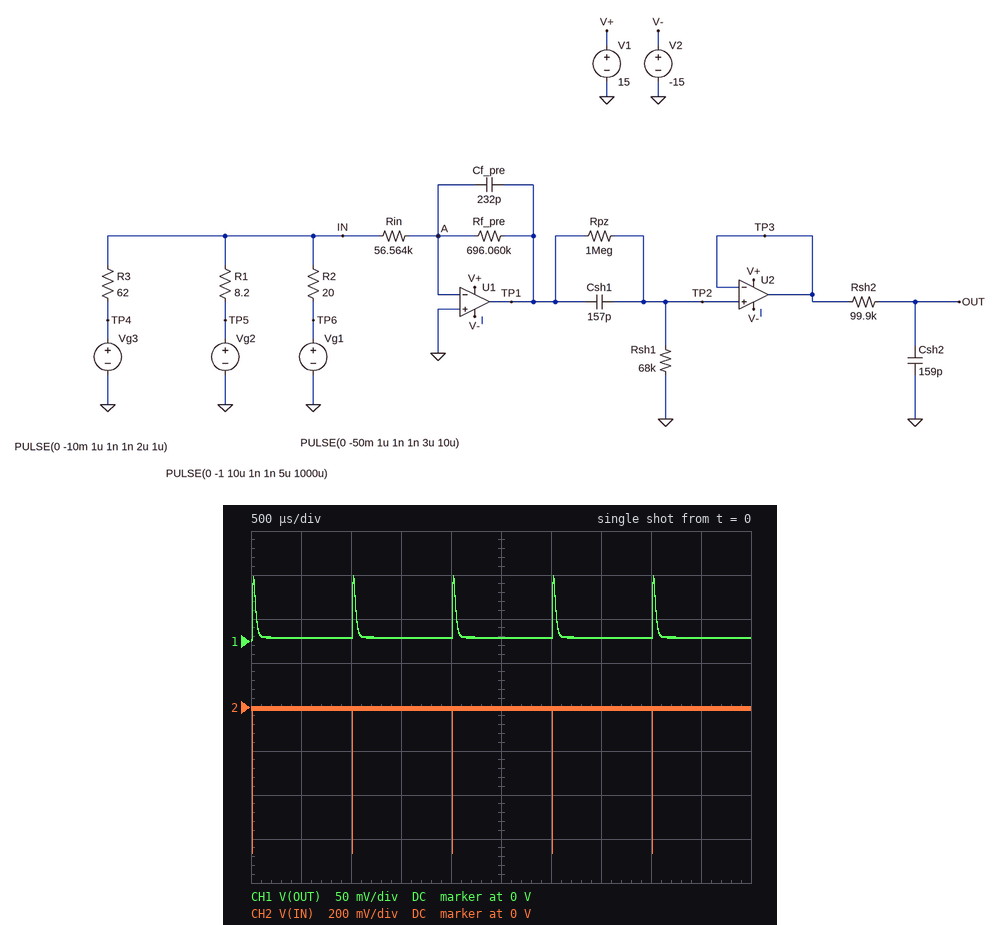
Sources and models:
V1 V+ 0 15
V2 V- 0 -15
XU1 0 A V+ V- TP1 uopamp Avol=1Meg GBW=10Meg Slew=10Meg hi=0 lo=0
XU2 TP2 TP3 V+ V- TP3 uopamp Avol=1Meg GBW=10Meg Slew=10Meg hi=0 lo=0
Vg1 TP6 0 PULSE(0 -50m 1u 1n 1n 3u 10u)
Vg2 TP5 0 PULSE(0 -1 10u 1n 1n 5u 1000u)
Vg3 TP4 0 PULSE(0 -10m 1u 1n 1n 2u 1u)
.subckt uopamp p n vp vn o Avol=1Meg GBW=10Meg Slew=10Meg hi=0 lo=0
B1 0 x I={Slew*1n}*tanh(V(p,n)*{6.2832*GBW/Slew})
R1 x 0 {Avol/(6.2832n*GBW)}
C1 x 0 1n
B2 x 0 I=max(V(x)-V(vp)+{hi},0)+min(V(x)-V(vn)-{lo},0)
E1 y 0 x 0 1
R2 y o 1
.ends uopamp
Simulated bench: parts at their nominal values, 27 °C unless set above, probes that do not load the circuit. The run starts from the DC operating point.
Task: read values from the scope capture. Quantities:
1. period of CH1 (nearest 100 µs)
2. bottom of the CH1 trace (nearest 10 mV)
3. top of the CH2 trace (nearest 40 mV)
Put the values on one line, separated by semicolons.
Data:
1.0 ms; 0 V; 0 V
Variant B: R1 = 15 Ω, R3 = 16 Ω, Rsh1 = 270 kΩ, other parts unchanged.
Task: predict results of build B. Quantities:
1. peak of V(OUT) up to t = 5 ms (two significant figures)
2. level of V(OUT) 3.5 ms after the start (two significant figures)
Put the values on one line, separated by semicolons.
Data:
92 mV; 20 mV
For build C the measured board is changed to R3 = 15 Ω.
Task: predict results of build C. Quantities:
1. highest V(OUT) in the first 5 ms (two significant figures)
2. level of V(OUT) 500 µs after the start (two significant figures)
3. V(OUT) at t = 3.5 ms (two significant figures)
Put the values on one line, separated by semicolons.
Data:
60 mV; 4.6 mV; 4.7 mV
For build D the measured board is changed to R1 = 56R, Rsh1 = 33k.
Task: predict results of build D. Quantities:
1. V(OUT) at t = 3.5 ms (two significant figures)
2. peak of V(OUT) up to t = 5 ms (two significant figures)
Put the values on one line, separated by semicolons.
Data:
4.2 mV; 19 mV
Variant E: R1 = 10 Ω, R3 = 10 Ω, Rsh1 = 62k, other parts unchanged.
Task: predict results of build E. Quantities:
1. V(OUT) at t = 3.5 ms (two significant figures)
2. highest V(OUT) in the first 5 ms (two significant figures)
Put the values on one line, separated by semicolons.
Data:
5.0 mV; 46 mV
